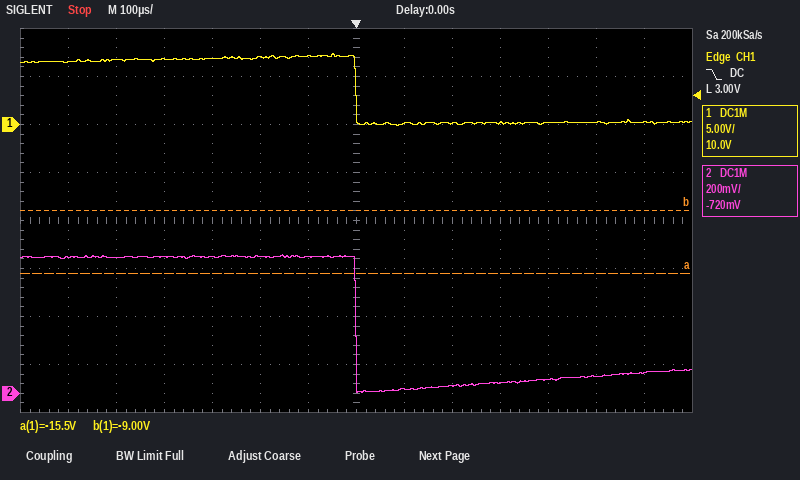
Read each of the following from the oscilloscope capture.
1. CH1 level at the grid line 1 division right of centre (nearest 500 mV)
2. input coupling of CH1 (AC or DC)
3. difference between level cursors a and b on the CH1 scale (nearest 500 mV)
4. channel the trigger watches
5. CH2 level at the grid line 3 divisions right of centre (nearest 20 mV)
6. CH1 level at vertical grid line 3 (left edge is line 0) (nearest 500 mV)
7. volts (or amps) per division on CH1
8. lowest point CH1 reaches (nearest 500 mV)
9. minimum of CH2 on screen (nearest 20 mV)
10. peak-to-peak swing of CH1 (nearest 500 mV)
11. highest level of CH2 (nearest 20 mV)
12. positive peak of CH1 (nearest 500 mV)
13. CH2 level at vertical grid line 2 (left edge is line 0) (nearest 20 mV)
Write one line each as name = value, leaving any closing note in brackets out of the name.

CH1 level at the grid line 1 division right of centre = 0.0 V
input coupling of CH1 = DC
difference between level cursors a and b on the CH1 scale = 6.5 V
channel the trigger watches = CH1
CH2 level at the grid line 3 divisions right of centre = 40 mV
CH1 level at vertical grid line 3 (left edge is line 0) = 7.0 V
volts (or amps) per division on CH1 = 5 V
lowest point CH1 reaches = 0.0 V
minimum of CH2 on screen = 0 mV
peak-to-peak swing of CH1 = 7.5 V
highest level of CH2 = 580 mV
positive peak of CH1 = 7.5 V
CH2 level at vertical grid line 2 (left edge is line 0) = 560 mV
